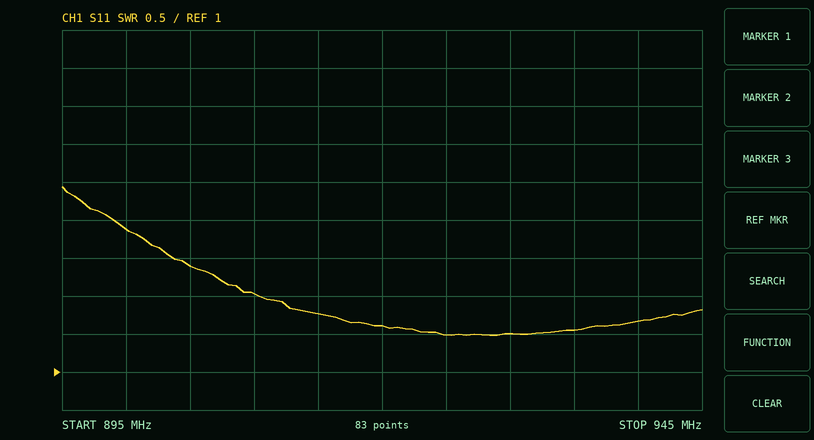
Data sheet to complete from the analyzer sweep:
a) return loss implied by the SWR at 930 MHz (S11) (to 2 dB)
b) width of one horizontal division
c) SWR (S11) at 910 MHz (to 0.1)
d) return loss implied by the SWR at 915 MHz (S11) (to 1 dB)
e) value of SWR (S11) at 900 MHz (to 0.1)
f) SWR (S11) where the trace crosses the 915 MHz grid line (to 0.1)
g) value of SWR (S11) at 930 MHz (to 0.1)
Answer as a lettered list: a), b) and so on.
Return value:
a) 14 dB
b) 5 MHz
c) 2.0
d) 11 dB
e) 2.9
f) 1.8
g) 1.5
